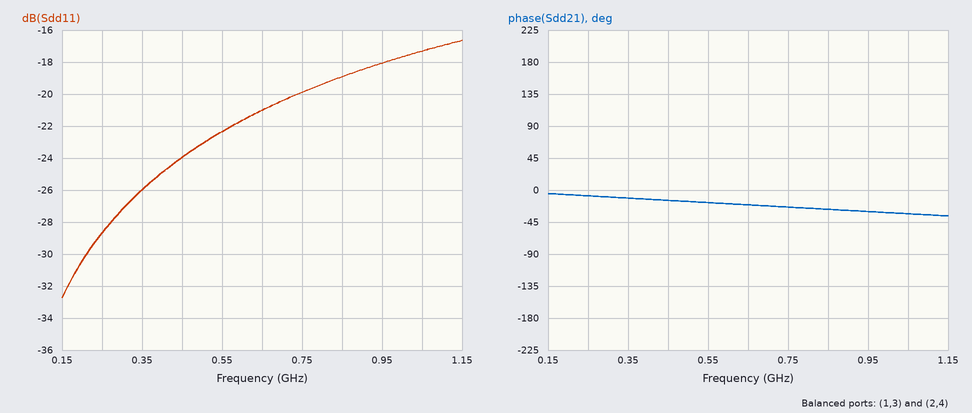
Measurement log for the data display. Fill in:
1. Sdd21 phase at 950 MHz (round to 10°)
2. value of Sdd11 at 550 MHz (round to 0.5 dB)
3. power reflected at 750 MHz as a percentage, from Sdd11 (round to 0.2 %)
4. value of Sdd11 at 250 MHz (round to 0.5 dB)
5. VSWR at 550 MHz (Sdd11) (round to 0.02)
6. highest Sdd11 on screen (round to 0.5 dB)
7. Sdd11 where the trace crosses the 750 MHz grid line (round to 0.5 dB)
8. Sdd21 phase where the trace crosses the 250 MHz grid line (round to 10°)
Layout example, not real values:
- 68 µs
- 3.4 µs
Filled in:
- -30°
- -22.5 dB
- 1.0 %
- -28.5 dB
- 1.16
- -16.5 dB
- -20.0 dB
- -10°
